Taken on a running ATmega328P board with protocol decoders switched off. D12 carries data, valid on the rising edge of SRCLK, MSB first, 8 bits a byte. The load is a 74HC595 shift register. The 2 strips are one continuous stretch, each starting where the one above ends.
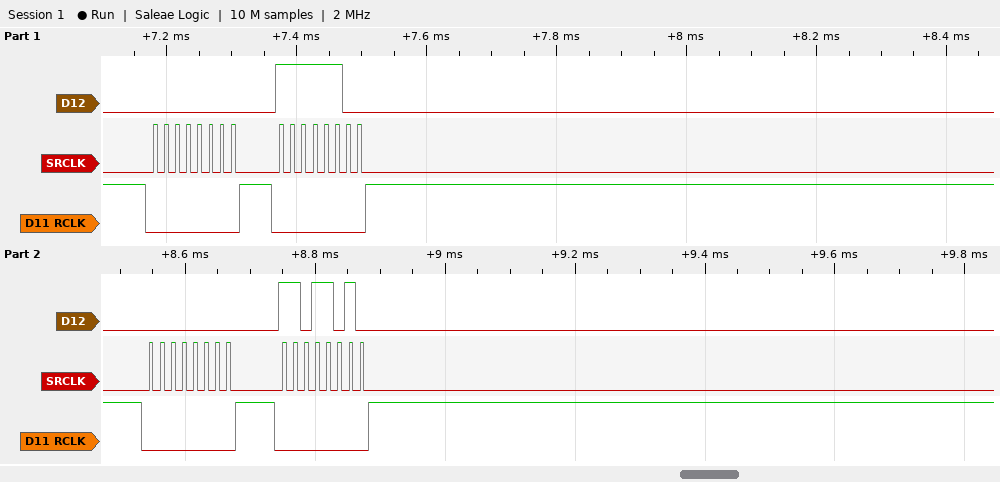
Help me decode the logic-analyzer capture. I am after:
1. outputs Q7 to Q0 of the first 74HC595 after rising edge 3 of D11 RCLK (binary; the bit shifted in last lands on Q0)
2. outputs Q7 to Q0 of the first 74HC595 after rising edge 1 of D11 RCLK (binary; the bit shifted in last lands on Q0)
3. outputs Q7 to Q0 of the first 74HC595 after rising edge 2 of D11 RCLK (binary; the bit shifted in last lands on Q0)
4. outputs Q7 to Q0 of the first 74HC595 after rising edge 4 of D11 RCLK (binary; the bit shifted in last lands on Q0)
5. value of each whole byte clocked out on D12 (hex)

00000000
00000000
11111100
11011010
0x00 0xFC 0x00 0xDA
